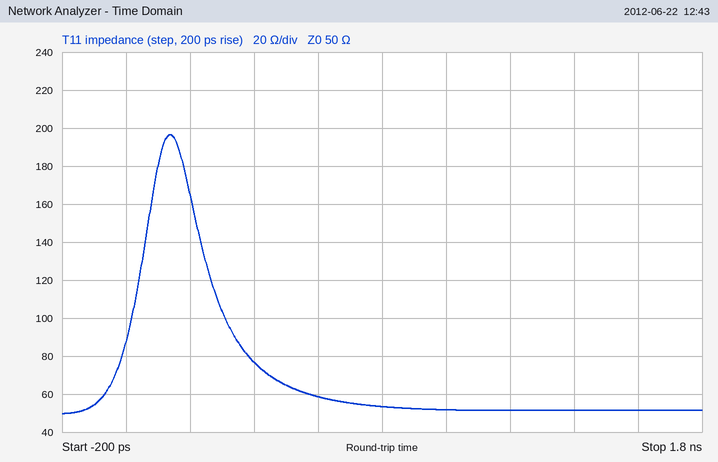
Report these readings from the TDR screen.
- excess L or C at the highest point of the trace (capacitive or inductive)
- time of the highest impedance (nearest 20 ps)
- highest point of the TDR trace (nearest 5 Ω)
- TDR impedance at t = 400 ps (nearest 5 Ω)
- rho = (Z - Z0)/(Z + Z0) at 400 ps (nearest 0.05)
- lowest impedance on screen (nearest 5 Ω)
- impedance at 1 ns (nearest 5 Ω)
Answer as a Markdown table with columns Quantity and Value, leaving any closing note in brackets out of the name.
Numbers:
| Quantity | Value |
|---|---|
| excess L or C at the highest point of the trace | inductive |
| time of the highest impedance | 140 ps |
| highest point of the TDR trace | 195 Ω |
| TDR impedance at t = 400 ps | 75 Ω |
| rho = (Z - Z0)/(Z + Z0) at 400 ps | +0.20 |
| lowest impedance on screen | 50 Ω |
| impedance at 1 ns | 50 Ω |
